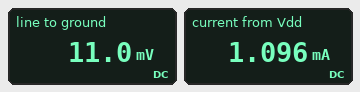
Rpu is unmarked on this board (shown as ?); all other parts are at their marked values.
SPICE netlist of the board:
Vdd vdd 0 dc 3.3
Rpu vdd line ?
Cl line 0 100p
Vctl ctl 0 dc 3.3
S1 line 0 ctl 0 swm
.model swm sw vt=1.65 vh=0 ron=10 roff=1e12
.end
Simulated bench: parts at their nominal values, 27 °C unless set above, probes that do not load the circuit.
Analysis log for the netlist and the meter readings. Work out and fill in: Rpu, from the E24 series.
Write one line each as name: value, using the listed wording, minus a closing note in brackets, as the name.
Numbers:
Rpu, from the E24 series: 3 kΩ
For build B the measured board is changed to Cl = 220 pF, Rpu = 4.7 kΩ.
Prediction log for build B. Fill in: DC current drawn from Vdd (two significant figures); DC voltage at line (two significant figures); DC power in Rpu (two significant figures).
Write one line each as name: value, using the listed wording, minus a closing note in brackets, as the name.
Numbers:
DC current drawn from Vdd: 700 µA
DC voltage at line: 7.0 mV
DC power in Rpu: 2.3 mW
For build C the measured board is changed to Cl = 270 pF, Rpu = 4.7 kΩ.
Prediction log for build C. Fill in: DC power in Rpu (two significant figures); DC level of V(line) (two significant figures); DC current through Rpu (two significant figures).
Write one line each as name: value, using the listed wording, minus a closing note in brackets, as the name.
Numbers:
DC power in Rpu: 2.3 mW
DC level of V(line): 7.0 mV
DC current through Rpu: 700 µA
